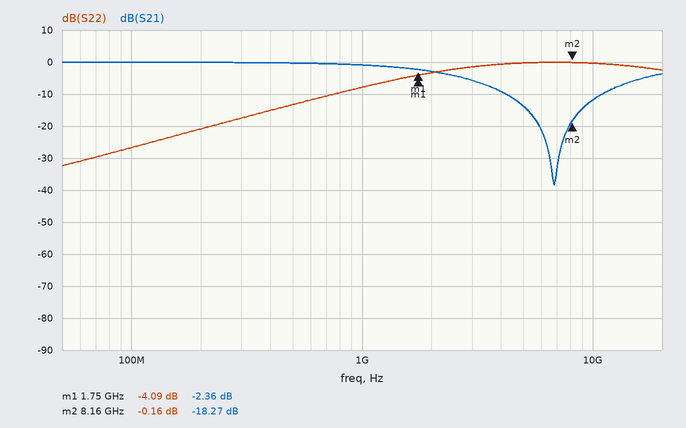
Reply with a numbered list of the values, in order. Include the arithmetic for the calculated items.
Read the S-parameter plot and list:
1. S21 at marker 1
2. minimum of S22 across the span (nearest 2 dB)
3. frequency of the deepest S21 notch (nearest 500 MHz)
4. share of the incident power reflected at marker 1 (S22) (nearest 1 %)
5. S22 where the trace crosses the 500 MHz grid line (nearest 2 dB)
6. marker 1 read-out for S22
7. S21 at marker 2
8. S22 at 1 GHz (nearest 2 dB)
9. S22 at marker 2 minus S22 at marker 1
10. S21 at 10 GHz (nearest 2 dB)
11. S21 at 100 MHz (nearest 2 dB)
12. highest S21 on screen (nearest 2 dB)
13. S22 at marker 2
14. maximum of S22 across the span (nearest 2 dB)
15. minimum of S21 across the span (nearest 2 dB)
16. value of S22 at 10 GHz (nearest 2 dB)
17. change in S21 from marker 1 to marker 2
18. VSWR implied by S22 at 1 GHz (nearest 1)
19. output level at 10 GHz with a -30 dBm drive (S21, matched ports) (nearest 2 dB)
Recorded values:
1. -2.36 dB
2. -32 dB
3. 7.0 GHz
4. 10^(-4.09/10) ≈ 39 %
5. -14 dB
6. -4.09 dB
7. -18.27 dB
8. -8 dB
9. -0.16 − (-4.09) = 3.93 dB
10. -12 dB
11. 0 dB
12. 0 dB
13. -0.16 dB
14. 0 dB
15. -38 dB
16. 0 dB
17. -18.27 − (-2.36) = -15.91 dB
18. |Γ| = 10^(-8/20) = 0.3981; VSWR = (1 + 0.3981)/(1 − 0.3981) ≈ 2
19. -30 dBm + (-12 dB) = -42 dBm
